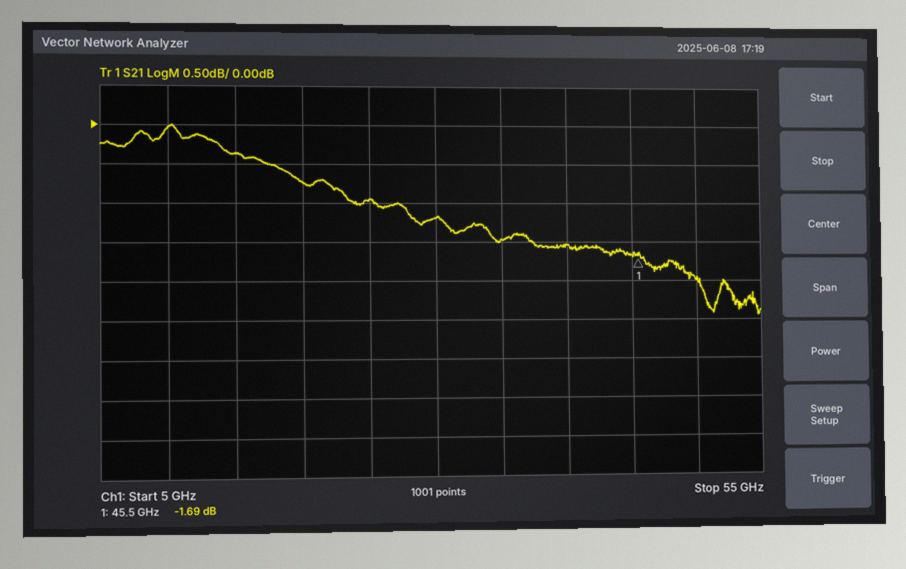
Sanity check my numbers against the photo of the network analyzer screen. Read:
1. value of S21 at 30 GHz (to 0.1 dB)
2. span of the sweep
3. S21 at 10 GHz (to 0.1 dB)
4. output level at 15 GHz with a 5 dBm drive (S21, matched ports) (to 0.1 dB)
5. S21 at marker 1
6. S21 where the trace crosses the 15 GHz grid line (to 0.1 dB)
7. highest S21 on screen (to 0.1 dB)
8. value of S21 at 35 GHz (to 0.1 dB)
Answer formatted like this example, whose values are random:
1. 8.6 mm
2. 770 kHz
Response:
1. -1.2 dB
2. 50 GHz
3. 0.0 dB
4. 4.6 dBm
5. -1.69 dB
6. -0.4 dB
7. 0.0 dB
8. -1.5 dB
